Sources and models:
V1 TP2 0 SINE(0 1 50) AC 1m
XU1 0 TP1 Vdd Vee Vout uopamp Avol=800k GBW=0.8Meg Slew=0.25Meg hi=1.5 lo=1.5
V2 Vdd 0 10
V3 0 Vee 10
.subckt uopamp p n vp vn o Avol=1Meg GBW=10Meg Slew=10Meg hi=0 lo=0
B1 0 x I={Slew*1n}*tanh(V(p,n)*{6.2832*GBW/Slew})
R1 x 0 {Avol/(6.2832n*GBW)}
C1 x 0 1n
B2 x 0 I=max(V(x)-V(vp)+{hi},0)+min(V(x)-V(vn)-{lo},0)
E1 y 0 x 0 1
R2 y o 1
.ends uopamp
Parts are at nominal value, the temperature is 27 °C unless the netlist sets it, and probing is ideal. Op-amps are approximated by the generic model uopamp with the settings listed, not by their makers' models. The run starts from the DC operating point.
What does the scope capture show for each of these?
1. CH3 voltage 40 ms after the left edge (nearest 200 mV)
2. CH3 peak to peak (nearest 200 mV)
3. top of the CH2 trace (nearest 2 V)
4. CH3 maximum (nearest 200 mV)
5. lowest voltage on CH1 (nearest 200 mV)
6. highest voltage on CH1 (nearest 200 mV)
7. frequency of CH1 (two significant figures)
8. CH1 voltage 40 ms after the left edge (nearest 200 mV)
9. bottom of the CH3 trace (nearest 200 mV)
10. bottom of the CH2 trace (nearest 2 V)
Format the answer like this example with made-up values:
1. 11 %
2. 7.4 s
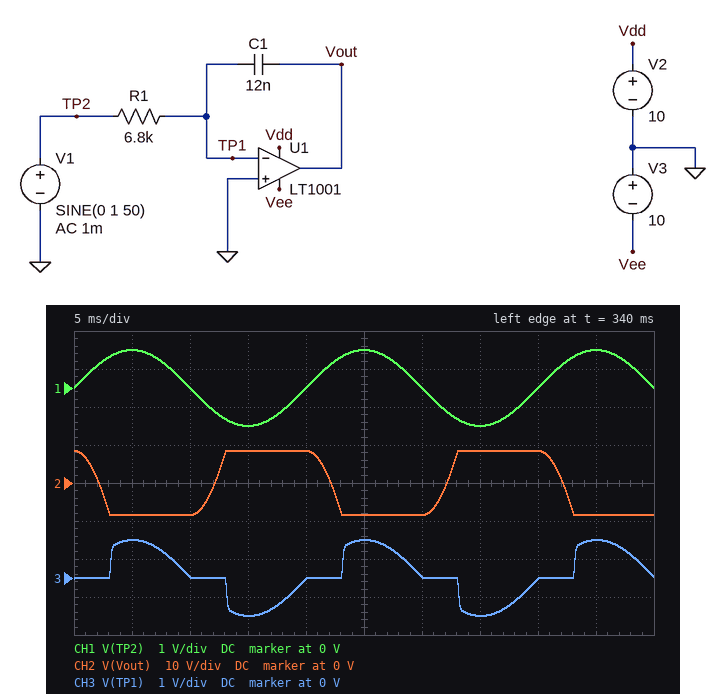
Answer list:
1. 0 V
2. 2.0 V
3. 8 V
4. 1.0 V
5. -1.0 V
6. 1.0 V
7. 50 Hz
8. 0 V
9. -1.0 V
10. -8 V
